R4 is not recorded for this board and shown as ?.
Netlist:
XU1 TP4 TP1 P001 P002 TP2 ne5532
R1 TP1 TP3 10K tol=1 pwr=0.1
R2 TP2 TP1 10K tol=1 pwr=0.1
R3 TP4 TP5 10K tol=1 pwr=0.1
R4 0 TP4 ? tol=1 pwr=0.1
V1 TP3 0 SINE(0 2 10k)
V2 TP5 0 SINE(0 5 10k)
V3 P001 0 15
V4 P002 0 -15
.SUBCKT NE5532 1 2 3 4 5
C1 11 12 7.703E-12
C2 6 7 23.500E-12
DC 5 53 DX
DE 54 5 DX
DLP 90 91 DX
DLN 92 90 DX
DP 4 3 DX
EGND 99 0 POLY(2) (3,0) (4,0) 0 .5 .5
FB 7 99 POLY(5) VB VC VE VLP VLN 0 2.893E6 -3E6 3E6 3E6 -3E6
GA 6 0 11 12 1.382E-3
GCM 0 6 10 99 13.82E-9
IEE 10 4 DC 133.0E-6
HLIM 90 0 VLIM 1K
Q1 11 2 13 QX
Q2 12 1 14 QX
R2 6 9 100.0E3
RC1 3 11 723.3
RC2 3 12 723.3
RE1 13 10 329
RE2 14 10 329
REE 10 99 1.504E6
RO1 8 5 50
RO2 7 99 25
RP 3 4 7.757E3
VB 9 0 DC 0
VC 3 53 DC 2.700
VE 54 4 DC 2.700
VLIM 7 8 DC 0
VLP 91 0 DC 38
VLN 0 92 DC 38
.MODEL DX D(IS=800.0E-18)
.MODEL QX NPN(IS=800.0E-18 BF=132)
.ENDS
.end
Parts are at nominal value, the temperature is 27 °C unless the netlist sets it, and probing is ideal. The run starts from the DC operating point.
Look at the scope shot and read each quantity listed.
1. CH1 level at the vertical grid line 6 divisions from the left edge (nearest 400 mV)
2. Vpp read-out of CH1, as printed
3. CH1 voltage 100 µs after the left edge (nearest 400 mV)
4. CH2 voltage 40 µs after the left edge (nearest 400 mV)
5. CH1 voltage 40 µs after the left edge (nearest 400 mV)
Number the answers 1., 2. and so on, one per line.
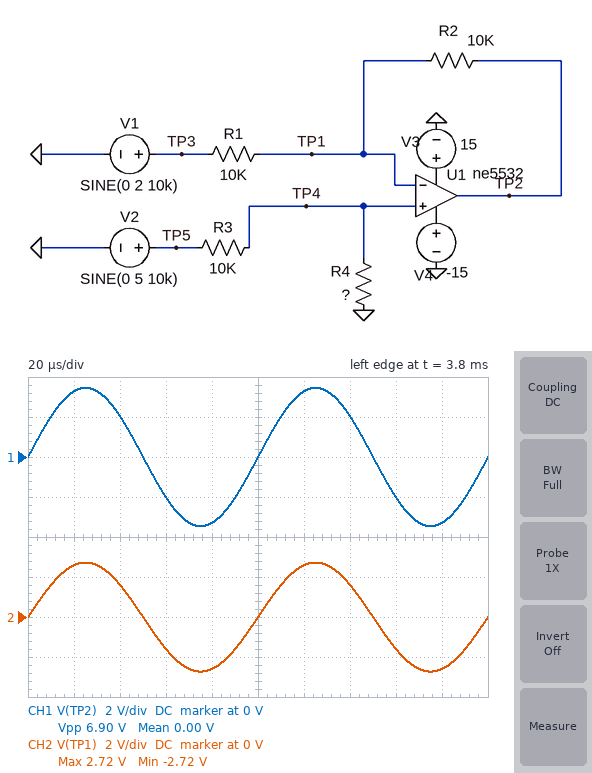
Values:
1. 3.2 V
2. 6.90 V
3. 0 V
4. 1.6 V
5. 2.0 V
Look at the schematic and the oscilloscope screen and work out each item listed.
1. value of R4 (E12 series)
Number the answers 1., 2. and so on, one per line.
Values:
1. 12 kΩ
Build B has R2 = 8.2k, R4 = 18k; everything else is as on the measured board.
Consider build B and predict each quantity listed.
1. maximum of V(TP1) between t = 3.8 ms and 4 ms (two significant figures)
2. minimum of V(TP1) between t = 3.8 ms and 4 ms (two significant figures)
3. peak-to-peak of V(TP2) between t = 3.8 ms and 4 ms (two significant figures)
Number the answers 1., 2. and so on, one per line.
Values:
1. 3.2 V
2. -3.2 V
3. 8.4 V
